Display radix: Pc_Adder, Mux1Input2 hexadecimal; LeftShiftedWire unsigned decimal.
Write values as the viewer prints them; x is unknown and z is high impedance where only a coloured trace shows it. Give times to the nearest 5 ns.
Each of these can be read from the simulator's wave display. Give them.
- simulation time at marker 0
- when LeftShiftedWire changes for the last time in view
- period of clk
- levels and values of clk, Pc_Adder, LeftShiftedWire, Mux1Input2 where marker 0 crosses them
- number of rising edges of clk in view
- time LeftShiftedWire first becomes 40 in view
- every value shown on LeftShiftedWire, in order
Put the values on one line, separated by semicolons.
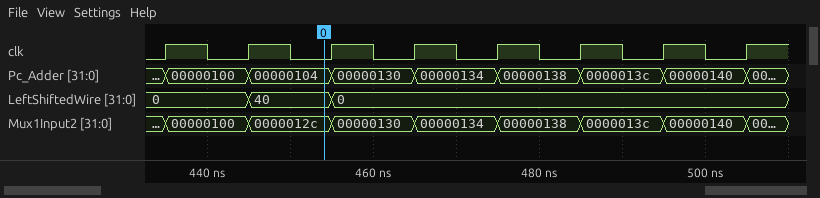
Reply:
455 ns; 455 ns; 10 ns; clk=0, Pc_Adder=00000104, LeftShiftedWire=40, Mux1Input2=0000012c; 8; 445 ns; 0, 40, 0
